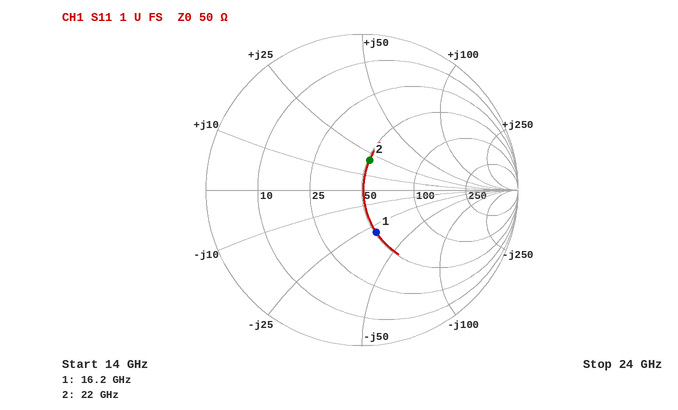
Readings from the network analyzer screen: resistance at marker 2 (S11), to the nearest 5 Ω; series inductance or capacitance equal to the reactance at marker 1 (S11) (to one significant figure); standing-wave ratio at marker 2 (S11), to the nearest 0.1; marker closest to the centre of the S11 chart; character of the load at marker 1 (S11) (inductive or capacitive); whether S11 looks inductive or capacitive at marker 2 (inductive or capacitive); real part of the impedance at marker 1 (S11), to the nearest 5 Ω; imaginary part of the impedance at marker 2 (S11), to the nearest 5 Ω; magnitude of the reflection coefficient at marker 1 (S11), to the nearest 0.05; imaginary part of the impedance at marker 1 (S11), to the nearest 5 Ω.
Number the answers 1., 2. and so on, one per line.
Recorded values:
1. 50 Ω
2. 300 fF
3. 1.5
4. marker 2
5. capacitive
6. inductive
7. 50 Ω
8. +20 Ω
9. 0.30
10. -30 Ω
